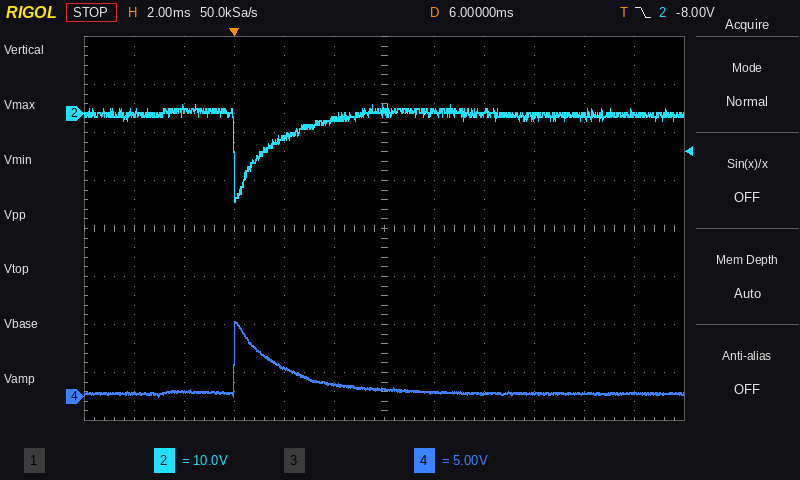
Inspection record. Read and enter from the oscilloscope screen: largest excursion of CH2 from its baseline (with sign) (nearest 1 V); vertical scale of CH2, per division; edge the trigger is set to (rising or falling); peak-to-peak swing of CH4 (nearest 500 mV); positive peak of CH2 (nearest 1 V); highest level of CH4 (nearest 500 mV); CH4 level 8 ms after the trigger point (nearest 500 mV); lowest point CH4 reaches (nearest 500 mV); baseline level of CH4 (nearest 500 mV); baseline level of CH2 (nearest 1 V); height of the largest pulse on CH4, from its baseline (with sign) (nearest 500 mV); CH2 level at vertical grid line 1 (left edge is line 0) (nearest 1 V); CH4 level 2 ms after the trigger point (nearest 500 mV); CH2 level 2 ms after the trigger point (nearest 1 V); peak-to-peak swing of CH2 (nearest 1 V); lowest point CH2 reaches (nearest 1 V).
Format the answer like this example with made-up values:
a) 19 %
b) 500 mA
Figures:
a) -18 V
b) 10 V
c) falling
d) 8.0 V
e) 2 V
f) 8.0 V
g) 500 mV
h) 0.0 V
i) 500 mV
j) 0 V
k) +7.5 V
l) 0 V
m) 3.0 V
n) -5 V
o) 20 V
p) -18 V
